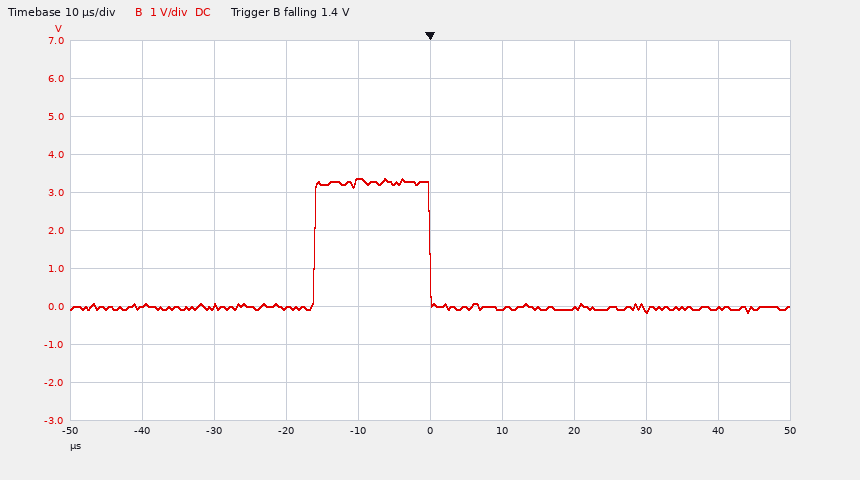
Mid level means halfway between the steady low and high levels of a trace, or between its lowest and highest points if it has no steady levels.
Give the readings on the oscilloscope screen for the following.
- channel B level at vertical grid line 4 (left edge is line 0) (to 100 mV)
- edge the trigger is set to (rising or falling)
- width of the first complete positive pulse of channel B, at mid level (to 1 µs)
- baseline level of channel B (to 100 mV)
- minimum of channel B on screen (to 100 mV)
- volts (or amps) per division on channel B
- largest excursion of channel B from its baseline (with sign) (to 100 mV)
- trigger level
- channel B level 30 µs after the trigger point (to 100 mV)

3.3 V
falling
16 µs
0.0 V
-200 mV
1 V
+3.4 V
1.4 V
-100 mV
